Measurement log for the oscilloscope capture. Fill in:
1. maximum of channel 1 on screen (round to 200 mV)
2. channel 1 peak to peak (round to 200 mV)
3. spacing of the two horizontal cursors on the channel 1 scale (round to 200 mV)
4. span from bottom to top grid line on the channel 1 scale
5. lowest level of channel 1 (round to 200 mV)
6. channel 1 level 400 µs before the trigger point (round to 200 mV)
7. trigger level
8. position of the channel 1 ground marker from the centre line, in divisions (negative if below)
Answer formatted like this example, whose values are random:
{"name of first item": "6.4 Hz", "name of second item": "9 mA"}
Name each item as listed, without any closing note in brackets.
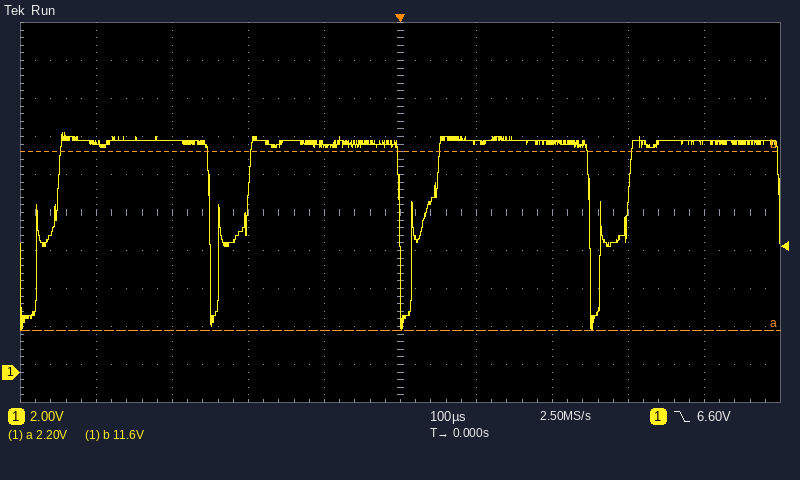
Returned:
{"maximum of channel 1 on screen": "12.6 V", "channel 1 peak to peak": "10.4 V", "spacing of the two horizontal cursors on the channel 1 scale": "9.4 V", "span from bottom to top grid line on the channel 1 scale": "20 V", "lowest level of channel 1": "2.2 V", "channel 1 level 400 µs before the trigger point": "12.0 V", "trigger level": "6.60 V", "position of the channel 1 ground marker from the centre line, in divisions": "-4.2 div"}
